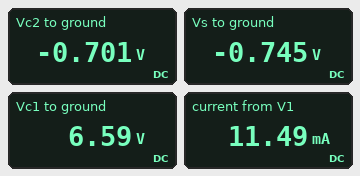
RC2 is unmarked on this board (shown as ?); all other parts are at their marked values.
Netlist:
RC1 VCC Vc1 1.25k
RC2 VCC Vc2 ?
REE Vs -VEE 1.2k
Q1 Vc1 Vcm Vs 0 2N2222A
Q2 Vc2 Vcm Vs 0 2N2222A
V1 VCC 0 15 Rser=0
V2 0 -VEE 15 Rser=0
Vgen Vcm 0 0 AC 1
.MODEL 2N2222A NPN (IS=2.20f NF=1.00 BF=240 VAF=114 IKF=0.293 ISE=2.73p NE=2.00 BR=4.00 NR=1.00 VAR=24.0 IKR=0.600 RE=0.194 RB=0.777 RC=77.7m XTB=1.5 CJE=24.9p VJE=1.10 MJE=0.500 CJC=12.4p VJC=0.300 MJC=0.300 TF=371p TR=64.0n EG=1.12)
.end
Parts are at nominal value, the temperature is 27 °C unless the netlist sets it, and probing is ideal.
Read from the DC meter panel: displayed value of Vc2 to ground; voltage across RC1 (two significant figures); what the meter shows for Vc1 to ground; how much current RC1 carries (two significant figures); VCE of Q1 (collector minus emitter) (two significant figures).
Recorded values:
-0.701 V
8.4 V
6.59 V
6.7 mA
7.3 V
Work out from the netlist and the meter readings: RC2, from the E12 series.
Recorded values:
3.3 kΩ
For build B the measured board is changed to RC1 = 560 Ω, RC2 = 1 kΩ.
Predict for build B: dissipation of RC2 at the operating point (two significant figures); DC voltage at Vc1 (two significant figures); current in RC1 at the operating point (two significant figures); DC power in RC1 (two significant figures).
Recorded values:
34 mW
12 V
6.0 mA
20 mW
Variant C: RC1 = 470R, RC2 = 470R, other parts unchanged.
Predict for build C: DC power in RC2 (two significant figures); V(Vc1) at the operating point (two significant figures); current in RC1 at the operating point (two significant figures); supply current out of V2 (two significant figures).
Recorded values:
16 mW
12 V
5.9 mA
12 mA
